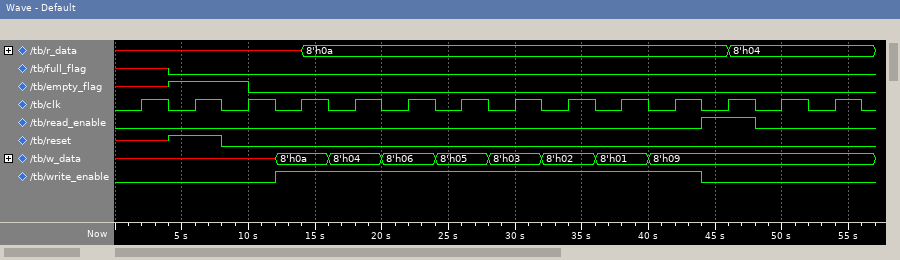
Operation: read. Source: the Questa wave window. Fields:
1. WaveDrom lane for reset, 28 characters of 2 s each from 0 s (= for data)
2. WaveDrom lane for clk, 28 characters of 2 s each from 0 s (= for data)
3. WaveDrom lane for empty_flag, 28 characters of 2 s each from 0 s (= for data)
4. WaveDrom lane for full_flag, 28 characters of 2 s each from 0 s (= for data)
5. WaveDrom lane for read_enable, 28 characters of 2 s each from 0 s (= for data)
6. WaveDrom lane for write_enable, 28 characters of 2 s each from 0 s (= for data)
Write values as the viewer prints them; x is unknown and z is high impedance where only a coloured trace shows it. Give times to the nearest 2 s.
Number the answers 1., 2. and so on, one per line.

1. {name: 'reset', wave: 'x.1.0.......................'}
2. {name: 'clk', wave: '0101010101010101010101010101'}
3. {name: 'empty_flag', wave: 'x.1..0......................'}
4. {name: 'full_flag', wave: 'x.0.........................'}
5. {name: 'read_enable', wave: '0.....................1.0...'}
6. {name: 'write_enable', wave: '0.....1...............0.....'}
